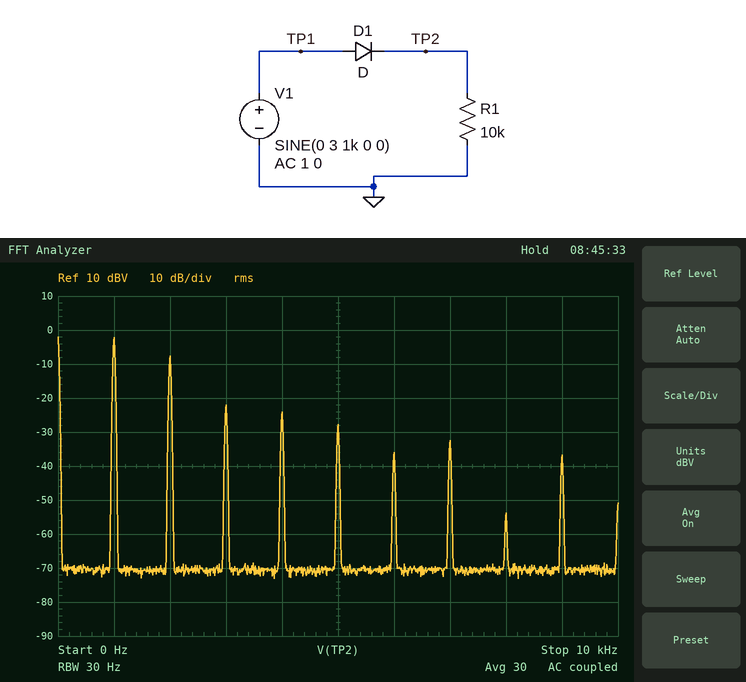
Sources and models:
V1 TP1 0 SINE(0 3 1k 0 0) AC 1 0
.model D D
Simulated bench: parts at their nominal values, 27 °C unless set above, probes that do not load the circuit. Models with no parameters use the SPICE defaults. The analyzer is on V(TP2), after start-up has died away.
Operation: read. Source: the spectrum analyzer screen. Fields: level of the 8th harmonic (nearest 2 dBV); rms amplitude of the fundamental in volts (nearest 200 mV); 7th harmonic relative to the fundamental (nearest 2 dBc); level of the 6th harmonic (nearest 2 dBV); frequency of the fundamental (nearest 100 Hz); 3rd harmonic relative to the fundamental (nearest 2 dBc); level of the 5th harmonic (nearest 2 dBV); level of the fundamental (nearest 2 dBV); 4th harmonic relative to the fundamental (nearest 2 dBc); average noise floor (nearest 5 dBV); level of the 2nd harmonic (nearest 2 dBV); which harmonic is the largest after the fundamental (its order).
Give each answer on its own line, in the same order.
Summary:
-54 dBV
800 mV
-30 dBc
-36 dBV
1.0 kHz
-20 dBc
-28 dBV
-2 dBV
-22 dBc
-70 dBV
-8 dBV
2
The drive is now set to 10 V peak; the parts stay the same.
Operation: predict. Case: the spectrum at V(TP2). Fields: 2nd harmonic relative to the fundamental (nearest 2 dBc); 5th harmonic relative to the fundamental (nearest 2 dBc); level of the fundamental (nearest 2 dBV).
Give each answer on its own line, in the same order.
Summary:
-6 dBc
-36 dBc
10 dBV
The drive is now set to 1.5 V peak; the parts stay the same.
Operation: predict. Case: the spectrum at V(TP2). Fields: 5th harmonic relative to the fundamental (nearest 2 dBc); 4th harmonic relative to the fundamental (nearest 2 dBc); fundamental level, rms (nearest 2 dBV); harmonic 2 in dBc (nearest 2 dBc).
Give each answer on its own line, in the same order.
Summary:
-22 dBc
-32 dBc
-12 dBV
-4 dBc
